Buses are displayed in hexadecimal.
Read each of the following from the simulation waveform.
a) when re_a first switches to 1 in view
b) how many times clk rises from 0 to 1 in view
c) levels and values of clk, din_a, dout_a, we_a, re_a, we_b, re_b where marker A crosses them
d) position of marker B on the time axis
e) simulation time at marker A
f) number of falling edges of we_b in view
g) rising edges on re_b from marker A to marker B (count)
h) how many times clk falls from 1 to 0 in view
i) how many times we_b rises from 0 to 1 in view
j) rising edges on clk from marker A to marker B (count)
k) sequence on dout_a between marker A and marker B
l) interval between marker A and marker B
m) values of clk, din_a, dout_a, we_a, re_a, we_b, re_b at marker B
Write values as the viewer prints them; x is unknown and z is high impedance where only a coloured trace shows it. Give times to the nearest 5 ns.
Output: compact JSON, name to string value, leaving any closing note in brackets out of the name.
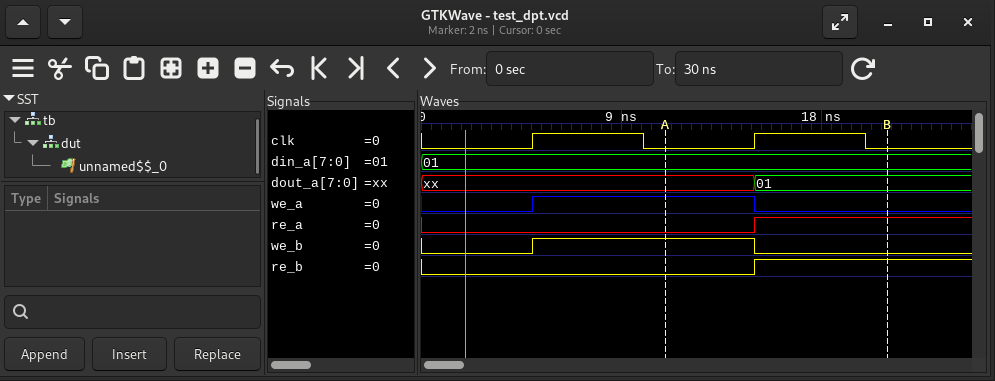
{"when re_a first switches to 1 in view": "15 ns", "how many times clk rises from 0 to 1 in view": "2", "levels and values of clk, din_a, dout_a, we_a, re_a, we_b, re_b where marker A crosses them": "clk=0, din_a=01, dout_a=xx, we_a=1, re_a=0, we_b=1, re_b=0", "position of marker B on the time axis": "20 ns", "simulation time at marker A": "10 ns", "number of falling edges of we_b in view": "1", "rising edges on re_b from marker A to marker B": "1", "how many times clk falls from 1 to 0 in view": "2", "how many times we_b rises from 0 to 1 in view": "1", "rising edges on clk from marker A to marker B": "1", "sequence on dout_a between marker A and marker B": "xx, 01", "interval between marker A and marker B": "10 ns", "values of clk, din_a, dout_a, we_a, re_a, we_b, re_b at marker B": "clk=0, din_a=01, dout_a=01, we_a=0, re_a=1, we_b=0, re_b=1"}
